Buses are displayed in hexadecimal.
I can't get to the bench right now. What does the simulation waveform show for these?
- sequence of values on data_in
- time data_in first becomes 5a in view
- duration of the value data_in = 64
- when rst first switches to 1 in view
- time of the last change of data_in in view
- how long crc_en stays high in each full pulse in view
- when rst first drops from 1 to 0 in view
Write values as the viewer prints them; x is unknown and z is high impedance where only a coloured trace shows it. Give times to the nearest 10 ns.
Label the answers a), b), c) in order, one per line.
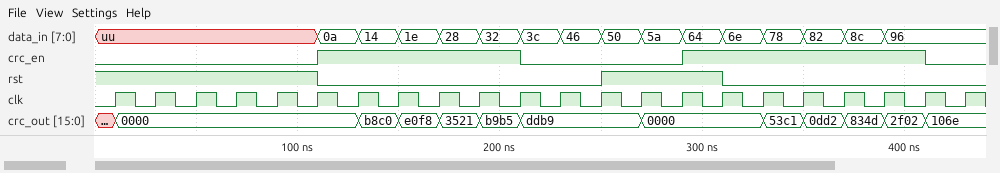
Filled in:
a) uu, 0a, 14, 1e, 28, 32, 3c, 46, 50, 5a, 64, 6e, 78, 82, 8c, 96
b) 270 ns
c) 20 ns
d) 250 ns
e) 390 ns
f) 100 ns, 120 ns
g) 110 ns
